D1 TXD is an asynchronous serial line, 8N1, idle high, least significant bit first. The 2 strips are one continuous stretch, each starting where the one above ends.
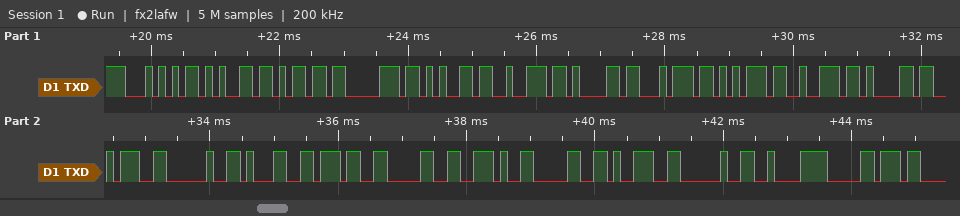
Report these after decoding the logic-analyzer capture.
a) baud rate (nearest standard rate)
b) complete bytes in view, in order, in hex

9600 baud
0x54 0x65 0x6D 0x70 0x65 0x72 0x61 0x74 0x75 0x72 0x61 0x3A 0x20 0x31 0x37 0x30 0x2E 0x30 0x39 0x20 0xC2 0xB0
